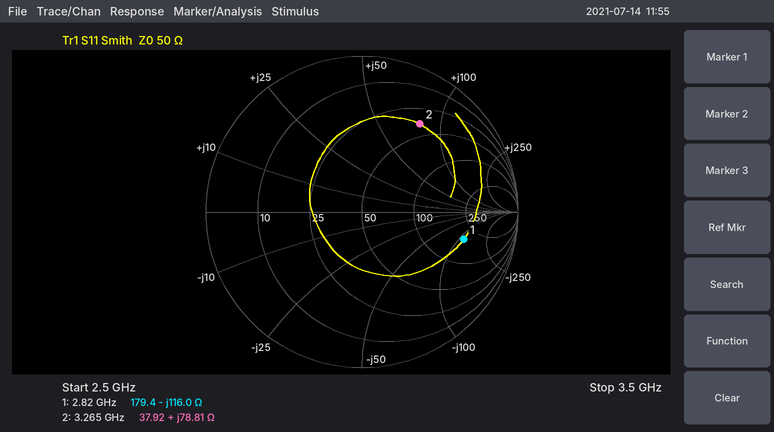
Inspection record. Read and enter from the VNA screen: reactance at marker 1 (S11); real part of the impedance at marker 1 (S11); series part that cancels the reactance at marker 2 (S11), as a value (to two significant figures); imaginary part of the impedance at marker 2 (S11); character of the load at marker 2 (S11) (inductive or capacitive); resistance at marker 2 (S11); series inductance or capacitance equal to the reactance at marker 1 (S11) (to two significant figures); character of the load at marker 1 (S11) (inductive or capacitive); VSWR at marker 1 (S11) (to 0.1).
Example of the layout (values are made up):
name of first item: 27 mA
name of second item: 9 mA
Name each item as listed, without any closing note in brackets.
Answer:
reactance at marker 1: -116.0 Ω
real part of the impedance at marker 1: 179.4 Ω
series part that cancels the reactance at marker 2 (S11), as a value: 620 fF
imaginary part of the impedance at marker 2: +78.81 Ω
character of the load at marker 2 (S11): inductive
resistance at marker 2: 37.92 Ω
series inductance or capacitance equal to the reactance at marker 1 (S11): 490 fF
character of the load at marker 1 (S11): capacitive
VSWR at marker 1 (S11): 5.2
